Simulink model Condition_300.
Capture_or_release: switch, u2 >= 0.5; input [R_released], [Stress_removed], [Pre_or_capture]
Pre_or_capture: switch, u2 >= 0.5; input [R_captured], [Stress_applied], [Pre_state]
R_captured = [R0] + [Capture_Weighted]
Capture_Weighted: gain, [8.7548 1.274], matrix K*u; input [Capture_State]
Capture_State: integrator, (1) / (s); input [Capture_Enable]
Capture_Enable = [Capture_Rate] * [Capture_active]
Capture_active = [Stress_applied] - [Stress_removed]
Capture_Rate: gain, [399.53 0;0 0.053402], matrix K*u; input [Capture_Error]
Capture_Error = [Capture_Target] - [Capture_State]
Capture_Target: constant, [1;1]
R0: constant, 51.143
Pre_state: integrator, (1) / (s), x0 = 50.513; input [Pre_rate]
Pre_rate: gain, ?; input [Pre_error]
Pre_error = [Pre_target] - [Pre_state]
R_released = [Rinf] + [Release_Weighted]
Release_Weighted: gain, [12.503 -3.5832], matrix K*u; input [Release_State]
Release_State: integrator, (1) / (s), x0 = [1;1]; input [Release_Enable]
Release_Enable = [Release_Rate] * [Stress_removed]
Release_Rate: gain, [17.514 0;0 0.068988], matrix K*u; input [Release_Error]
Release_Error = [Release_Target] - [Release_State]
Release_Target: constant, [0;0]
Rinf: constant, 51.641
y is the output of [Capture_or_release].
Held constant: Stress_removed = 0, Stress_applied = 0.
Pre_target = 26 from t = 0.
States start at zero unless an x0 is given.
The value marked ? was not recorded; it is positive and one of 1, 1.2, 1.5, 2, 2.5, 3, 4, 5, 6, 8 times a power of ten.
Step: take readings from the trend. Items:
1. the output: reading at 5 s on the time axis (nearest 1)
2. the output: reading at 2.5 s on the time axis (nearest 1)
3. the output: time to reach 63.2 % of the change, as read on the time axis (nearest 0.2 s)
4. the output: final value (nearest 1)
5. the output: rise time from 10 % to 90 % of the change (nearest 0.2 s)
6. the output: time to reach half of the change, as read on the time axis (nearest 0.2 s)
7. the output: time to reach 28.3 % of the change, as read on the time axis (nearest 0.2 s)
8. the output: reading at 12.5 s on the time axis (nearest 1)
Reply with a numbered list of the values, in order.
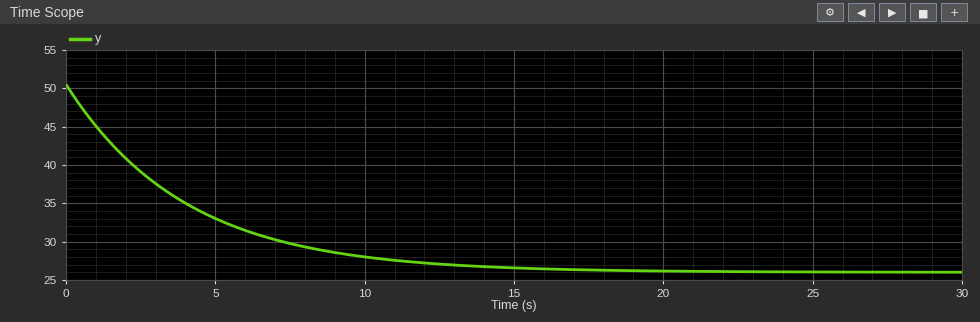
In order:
1. 33
2. 39
3. 4.0 s
4. 26
5. 8.8 s
6. 2.8 s
7. 1.4 s
8. 27
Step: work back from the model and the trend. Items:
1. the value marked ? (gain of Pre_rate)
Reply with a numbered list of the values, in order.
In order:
1. 0.25
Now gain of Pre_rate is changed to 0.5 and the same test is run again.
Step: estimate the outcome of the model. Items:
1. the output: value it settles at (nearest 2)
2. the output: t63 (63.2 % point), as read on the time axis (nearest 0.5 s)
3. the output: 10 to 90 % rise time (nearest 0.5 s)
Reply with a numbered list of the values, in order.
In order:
1. 26
2. 2.0 s
3. 4.5 s
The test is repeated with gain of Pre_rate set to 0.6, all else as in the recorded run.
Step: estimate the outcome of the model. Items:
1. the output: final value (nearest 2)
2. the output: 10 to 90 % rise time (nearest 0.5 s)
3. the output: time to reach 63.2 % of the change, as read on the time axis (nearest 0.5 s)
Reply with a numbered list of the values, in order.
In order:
1. 26
2. 3.5 s
3. 1.5 s
